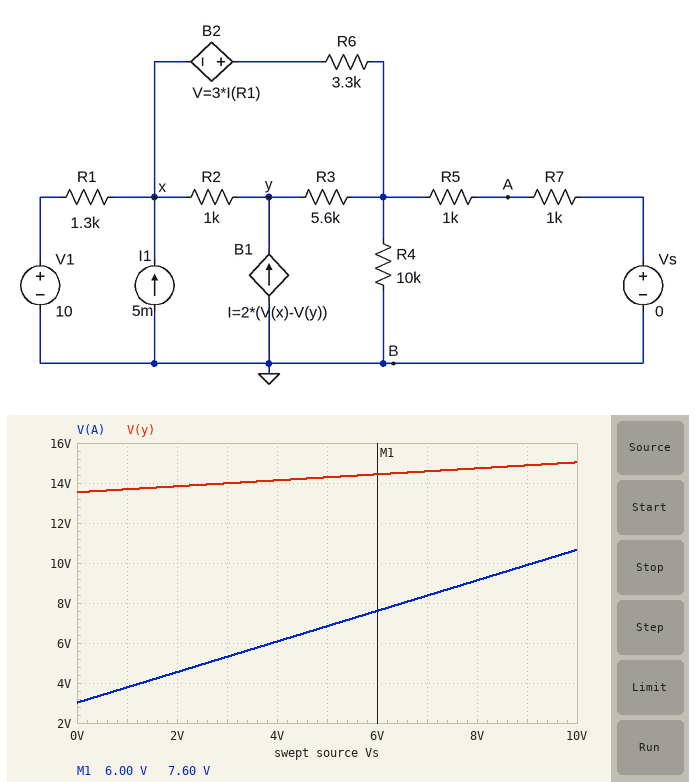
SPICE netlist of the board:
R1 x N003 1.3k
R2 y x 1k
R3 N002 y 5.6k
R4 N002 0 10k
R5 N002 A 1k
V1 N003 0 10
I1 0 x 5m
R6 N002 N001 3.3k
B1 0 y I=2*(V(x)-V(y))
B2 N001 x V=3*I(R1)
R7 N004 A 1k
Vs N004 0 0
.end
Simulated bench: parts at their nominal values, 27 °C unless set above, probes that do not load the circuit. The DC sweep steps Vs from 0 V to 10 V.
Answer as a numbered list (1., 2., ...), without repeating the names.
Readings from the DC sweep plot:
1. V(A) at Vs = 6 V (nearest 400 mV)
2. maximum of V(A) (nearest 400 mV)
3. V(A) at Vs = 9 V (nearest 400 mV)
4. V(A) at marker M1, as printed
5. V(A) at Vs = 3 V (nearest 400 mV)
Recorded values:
1. 7.6 V
2. 10.8 V
3. 10.0 V
4. 7.60 V
5. 5.2 V
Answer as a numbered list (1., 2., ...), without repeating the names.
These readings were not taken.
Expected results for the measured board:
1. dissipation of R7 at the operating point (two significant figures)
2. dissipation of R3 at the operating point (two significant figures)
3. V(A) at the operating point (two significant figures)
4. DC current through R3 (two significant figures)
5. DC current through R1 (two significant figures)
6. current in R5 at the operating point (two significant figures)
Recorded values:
1. 9.1 mW
2. 10 mW
3. 3.0 V
4. 1.3 mA
5. 2.7 mA
6. 3.0 mA
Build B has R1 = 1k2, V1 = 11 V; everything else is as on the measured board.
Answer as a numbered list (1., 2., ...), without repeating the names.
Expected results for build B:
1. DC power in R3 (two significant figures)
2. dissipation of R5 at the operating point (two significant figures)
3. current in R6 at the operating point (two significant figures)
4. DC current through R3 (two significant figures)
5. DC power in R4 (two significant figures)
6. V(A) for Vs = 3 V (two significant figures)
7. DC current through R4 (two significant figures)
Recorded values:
1. 11 mW
2. 9.9 mW
3. 2.4 mA
4. 1.4 mA
5. 4.0 mW
6. 5.4 V
7. 630 µA
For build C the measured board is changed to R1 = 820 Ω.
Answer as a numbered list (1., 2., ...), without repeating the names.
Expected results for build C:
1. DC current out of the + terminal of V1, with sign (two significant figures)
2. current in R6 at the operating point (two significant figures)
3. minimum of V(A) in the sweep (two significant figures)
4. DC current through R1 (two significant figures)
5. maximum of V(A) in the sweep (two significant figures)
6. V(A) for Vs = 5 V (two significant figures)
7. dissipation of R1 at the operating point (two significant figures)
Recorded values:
1. -2.9 mA
2. 2.1 mA
3. 2.8 V
4. 2.9 mA
5. 10 V
6. 6.5 V
7. 7.0 mW
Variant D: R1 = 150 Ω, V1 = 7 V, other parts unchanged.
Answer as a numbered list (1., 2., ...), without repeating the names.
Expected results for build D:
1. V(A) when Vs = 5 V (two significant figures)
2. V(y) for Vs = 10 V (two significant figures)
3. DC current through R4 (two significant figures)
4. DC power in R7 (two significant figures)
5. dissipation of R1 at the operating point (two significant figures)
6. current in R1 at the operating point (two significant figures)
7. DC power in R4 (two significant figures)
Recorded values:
1. 5.4 V
2. 7.8 V
3. 340 µA
4. 2.8 mW
5. 2.1 mW
6. 3.7 mA
7. 1.1 mW
